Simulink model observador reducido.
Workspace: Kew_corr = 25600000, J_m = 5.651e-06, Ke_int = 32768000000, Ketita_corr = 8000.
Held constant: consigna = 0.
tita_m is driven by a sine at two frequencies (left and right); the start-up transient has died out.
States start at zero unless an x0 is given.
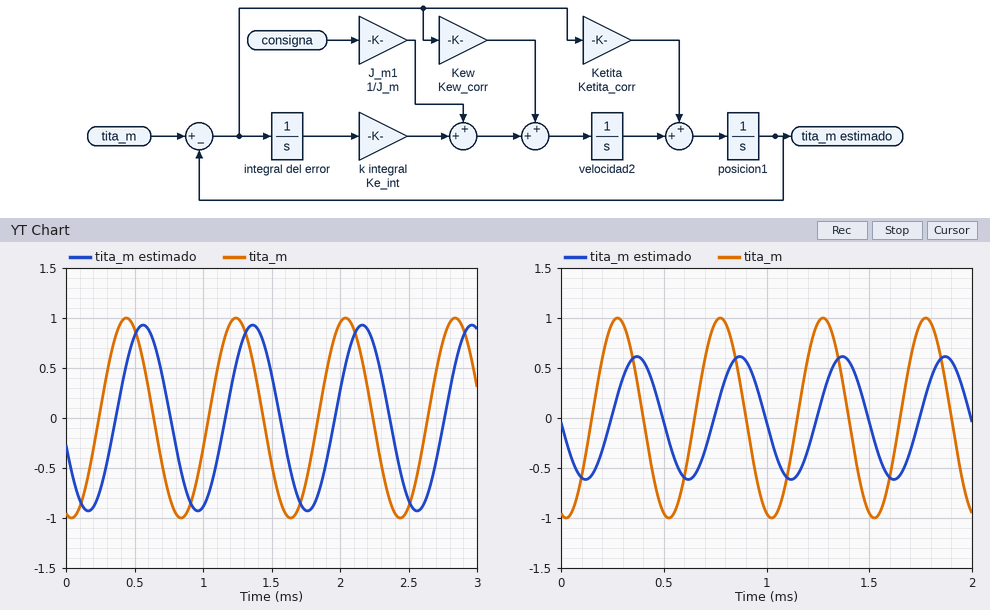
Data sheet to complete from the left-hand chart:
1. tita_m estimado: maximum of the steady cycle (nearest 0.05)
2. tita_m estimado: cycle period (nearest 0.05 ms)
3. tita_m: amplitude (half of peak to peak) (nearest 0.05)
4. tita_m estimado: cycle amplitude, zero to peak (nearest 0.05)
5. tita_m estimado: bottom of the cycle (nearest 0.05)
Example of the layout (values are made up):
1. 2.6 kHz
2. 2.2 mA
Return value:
1. 0.95
2. 0.80 ms
3. 1.00
4. 0.95
5. -0.95
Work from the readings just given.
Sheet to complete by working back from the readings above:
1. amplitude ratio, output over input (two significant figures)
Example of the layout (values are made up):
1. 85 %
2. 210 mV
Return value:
1. 0.95
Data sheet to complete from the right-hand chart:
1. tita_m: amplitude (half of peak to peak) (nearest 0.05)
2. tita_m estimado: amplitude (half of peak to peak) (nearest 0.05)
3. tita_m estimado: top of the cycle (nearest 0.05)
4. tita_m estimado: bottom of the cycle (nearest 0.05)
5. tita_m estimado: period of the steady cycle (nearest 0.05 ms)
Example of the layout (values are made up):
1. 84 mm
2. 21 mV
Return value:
1. 1.00
2. 0.60
3. 0.60
4. -0.60
5. 0.50 ms
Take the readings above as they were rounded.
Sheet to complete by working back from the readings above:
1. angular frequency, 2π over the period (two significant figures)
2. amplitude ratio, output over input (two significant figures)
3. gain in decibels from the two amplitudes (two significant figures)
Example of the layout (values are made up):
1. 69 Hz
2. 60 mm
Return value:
1. 13 rad/ms
2. 0.60
3. -4.4 dB
